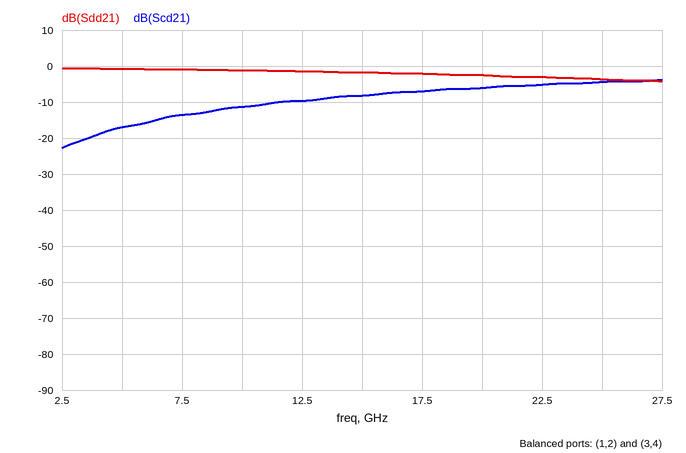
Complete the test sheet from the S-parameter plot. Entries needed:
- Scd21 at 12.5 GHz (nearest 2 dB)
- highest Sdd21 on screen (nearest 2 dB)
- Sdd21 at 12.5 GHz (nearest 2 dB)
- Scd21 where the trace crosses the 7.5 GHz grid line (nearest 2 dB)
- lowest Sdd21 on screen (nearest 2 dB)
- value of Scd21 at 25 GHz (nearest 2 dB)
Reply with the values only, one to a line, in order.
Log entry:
-10 dB
0 dB
-2 dB
-14 dB
-4 dB
-4 dB
